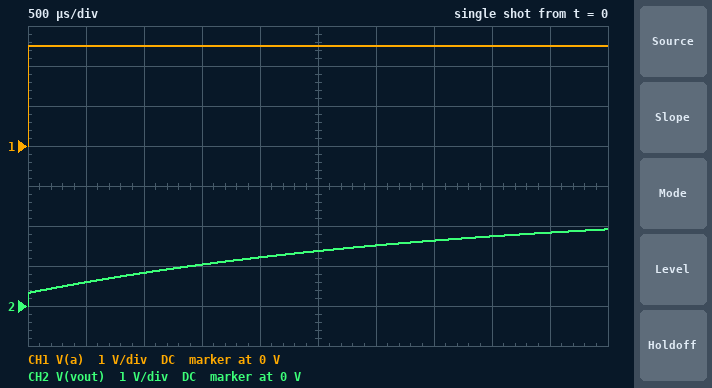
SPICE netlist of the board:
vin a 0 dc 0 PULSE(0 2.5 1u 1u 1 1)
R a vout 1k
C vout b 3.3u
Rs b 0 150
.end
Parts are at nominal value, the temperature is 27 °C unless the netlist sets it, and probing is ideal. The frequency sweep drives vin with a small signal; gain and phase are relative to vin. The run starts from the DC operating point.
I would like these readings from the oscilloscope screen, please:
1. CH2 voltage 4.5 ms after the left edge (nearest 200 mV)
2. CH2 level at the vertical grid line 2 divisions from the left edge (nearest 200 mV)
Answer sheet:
1.8 V
800 mV
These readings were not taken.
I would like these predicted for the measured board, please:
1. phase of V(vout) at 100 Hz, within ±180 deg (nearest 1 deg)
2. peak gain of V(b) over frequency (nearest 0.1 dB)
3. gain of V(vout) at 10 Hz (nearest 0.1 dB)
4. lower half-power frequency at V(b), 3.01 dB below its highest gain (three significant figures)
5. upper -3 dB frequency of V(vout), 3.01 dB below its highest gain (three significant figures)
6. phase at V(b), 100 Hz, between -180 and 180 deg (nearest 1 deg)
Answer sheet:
-50 deg
-17.7 dB
-0.2 dB
41.9 Hz
42.7 Hz
23 deg
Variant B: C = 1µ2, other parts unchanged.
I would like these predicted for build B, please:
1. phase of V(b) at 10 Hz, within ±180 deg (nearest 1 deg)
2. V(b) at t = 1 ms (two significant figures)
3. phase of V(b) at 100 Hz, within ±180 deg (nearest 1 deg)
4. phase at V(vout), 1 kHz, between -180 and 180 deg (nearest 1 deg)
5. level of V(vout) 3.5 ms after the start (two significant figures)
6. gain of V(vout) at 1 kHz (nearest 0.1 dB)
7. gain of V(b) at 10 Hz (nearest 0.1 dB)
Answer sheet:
85 deg
160 mV
49 deg
-35 deg
2.3 V
-15.2 dB
-39.0 dB
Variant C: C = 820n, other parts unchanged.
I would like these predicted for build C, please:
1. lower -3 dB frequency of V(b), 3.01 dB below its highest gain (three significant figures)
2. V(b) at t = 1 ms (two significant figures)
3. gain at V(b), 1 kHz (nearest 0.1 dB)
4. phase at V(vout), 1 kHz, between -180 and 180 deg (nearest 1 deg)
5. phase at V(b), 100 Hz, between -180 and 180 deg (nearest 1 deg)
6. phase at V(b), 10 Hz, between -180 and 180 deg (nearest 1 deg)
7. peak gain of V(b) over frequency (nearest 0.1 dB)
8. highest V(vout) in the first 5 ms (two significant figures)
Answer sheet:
169 Hz
110 mV
-17.8 dB
-43 deg
59 deg
87 deg
-17.7 dB
2.5 V
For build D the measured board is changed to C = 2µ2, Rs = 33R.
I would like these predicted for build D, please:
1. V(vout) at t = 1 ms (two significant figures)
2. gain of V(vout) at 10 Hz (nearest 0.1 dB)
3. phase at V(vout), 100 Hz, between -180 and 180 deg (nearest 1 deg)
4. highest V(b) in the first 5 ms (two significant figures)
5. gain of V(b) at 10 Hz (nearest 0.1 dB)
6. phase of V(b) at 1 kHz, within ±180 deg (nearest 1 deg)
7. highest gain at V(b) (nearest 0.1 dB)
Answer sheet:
940 mV
-0.1 dB
-52 deg
80 mV
-46.9 dB
4 deg
-29.9 dB
